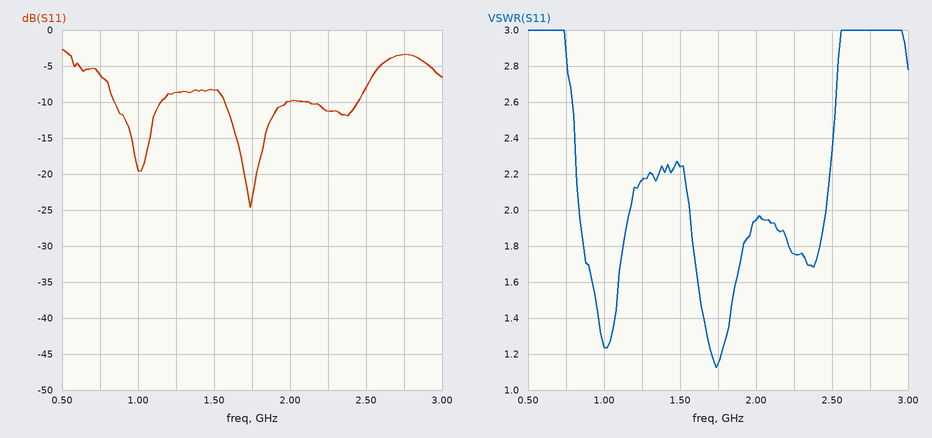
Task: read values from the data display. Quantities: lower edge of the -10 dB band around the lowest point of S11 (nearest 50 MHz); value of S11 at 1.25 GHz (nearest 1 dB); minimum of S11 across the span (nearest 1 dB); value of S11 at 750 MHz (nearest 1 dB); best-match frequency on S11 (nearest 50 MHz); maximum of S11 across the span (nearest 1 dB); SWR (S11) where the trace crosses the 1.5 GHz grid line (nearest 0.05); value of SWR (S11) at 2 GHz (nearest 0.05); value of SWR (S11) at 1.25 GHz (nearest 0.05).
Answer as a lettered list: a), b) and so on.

a) 1.55 GHz
b) -9 dB
c) -25 dB
d) -6 dB
e) 1.75 GHz
f) -3 dB
g) 2.25
h) 1.95
i) 2.15
